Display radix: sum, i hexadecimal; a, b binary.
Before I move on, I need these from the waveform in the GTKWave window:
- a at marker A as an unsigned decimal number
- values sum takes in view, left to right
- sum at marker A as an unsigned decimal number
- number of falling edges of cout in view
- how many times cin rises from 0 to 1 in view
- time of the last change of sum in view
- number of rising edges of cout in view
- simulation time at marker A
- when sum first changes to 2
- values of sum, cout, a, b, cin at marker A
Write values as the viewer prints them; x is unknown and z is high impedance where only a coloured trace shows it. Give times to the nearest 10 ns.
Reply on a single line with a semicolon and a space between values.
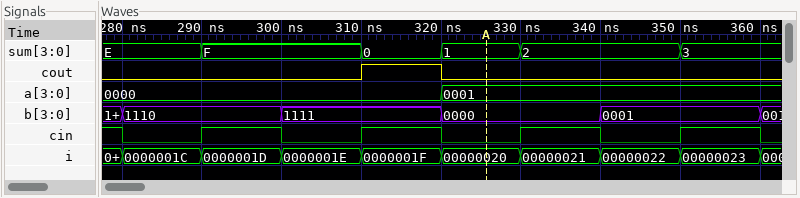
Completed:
1; E, F, 0, 1, 2, 3; 1; 1; 4; 350 ns; 1; 330 ns; 330 ns; sum=1, cout=0, a=0001, b=0000, cin=0
